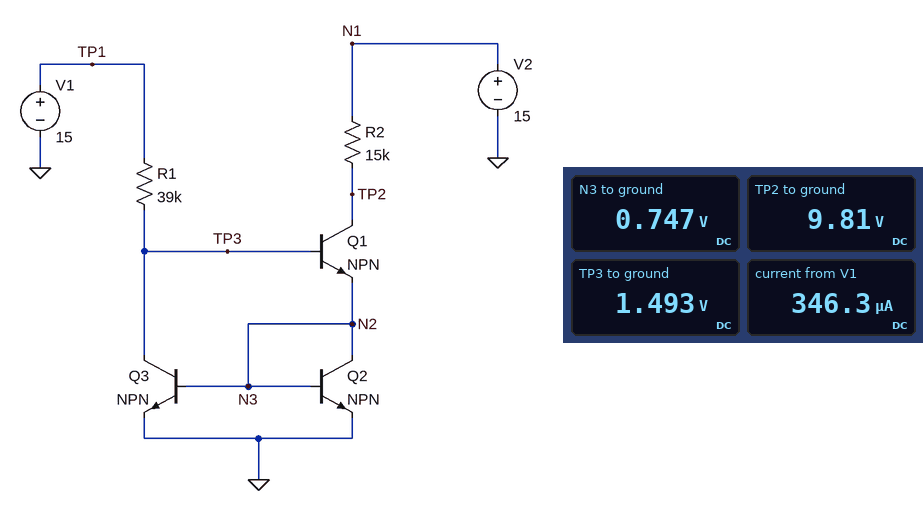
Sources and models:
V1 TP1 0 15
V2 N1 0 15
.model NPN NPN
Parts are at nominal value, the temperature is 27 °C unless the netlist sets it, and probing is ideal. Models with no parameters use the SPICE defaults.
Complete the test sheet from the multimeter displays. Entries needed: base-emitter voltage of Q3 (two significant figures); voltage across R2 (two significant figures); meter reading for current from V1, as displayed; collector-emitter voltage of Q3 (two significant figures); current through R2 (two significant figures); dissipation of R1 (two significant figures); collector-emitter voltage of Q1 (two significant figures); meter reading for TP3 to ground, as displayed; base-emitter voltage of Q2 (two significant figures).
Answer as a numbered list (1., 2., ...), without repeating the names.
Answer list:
1. 750 mV
2. 5.2 V
3. 346.3 µA
4. 1.5 V
5. 350 µA
6. 4.7 mW
7. 9.1 V
8. 1.493 V
9. 750 mV
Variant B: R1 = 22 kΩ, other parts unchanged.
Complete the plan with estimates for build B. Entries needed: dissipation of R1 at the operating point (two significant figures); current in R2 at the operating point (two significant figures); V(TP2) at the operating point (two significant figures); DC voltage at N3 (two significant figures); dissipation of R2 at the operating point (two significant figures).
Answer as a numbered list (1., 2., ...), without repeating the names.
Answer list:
1. 8.3 mW
2. 610 µA
3. 5.8 V
4. 760 mV
5. 5.6 mW
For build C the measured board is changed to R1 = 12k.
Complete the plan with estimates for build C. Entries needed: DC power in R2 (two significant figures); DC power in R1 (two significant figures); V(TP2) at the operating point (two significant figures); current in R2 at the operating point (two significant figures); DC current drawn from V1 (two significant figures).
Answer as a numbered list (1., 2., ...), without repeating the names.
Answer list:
1. 13 mW
2. 15 mW
3. 840 mV
4. 940 µA
5. 1.1 mA
